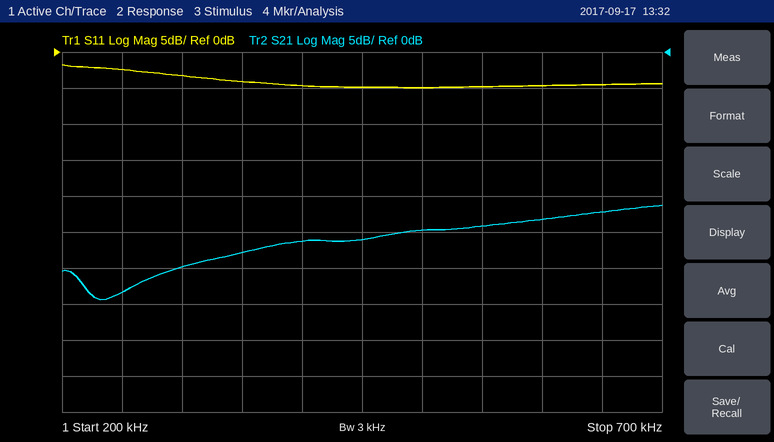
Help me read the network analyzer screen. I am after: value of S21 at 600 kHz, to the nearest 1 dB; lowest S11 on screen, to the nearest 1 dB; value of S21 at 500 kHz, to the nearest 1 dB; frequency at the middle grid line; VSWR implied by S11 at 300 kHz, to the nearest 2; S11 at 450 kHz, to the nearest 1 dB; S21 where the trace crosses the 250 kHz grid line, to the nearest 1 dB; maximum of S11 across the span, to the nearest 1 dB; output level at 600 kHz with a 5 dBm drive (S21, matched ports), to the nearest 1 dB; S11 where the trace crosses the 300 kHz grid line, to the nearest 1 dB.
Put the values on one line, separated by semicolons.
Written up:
-23 dB; -5 dB; -25 dB; 450 kHz; 6; -5 dB; -33 dB; -2 dB; -18 dBm; -3 dB
